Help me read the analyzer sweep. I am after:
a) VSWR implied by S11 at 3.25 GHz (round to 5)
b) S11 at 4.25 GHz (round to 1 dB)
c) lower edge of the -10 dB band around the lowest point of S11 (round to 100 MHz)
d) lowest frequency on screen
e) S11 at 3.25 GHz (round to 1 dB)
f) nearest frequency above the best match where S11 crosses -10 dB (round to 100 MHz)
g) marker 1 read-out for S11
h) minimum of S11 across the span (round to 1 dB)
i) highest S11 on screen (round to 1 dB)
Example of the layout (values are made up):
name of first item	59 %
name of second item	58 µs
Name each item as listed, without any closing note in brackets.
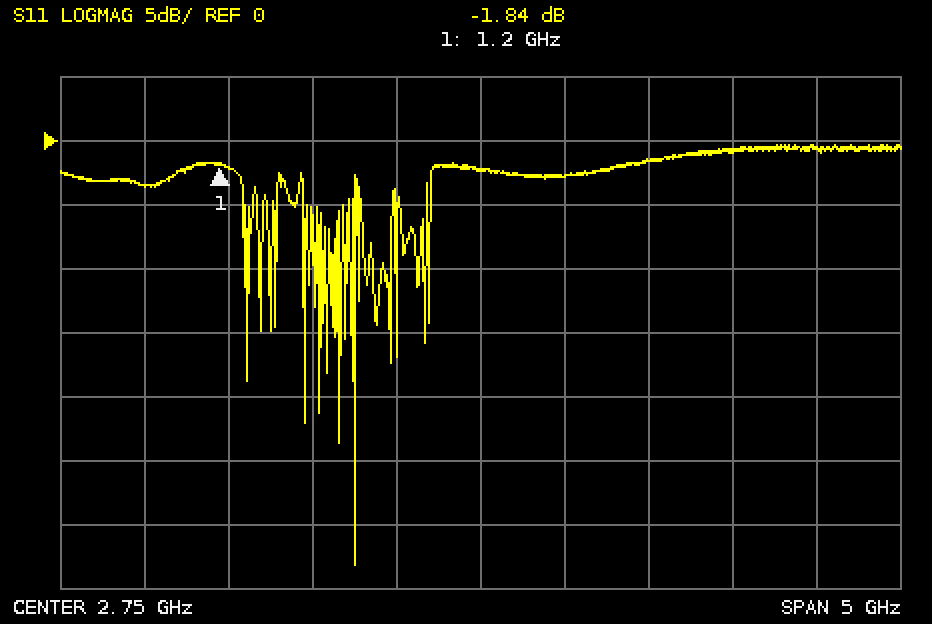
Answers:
VSWR implied by S11 at 3.25 GHz	5
S11 at 4.25 GHz	-1 dB
lower edge of the -10 dB band around the lowest point of S11	2.0 GHz
lowest frequency on screen	250 MHz
S11 at 3.25 GHz	-3 dB
nearest frequency above the best match where S11 crosses -10 dB	2.0 GHz
marker 1 read-out for S11	-1.84 dB
minimum of S11 across the span	-33 dB
highest S11 on screen	0 dB
